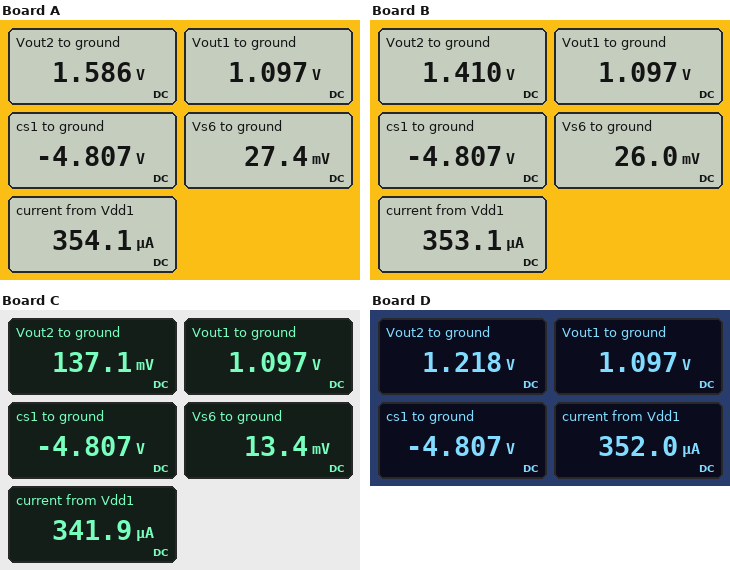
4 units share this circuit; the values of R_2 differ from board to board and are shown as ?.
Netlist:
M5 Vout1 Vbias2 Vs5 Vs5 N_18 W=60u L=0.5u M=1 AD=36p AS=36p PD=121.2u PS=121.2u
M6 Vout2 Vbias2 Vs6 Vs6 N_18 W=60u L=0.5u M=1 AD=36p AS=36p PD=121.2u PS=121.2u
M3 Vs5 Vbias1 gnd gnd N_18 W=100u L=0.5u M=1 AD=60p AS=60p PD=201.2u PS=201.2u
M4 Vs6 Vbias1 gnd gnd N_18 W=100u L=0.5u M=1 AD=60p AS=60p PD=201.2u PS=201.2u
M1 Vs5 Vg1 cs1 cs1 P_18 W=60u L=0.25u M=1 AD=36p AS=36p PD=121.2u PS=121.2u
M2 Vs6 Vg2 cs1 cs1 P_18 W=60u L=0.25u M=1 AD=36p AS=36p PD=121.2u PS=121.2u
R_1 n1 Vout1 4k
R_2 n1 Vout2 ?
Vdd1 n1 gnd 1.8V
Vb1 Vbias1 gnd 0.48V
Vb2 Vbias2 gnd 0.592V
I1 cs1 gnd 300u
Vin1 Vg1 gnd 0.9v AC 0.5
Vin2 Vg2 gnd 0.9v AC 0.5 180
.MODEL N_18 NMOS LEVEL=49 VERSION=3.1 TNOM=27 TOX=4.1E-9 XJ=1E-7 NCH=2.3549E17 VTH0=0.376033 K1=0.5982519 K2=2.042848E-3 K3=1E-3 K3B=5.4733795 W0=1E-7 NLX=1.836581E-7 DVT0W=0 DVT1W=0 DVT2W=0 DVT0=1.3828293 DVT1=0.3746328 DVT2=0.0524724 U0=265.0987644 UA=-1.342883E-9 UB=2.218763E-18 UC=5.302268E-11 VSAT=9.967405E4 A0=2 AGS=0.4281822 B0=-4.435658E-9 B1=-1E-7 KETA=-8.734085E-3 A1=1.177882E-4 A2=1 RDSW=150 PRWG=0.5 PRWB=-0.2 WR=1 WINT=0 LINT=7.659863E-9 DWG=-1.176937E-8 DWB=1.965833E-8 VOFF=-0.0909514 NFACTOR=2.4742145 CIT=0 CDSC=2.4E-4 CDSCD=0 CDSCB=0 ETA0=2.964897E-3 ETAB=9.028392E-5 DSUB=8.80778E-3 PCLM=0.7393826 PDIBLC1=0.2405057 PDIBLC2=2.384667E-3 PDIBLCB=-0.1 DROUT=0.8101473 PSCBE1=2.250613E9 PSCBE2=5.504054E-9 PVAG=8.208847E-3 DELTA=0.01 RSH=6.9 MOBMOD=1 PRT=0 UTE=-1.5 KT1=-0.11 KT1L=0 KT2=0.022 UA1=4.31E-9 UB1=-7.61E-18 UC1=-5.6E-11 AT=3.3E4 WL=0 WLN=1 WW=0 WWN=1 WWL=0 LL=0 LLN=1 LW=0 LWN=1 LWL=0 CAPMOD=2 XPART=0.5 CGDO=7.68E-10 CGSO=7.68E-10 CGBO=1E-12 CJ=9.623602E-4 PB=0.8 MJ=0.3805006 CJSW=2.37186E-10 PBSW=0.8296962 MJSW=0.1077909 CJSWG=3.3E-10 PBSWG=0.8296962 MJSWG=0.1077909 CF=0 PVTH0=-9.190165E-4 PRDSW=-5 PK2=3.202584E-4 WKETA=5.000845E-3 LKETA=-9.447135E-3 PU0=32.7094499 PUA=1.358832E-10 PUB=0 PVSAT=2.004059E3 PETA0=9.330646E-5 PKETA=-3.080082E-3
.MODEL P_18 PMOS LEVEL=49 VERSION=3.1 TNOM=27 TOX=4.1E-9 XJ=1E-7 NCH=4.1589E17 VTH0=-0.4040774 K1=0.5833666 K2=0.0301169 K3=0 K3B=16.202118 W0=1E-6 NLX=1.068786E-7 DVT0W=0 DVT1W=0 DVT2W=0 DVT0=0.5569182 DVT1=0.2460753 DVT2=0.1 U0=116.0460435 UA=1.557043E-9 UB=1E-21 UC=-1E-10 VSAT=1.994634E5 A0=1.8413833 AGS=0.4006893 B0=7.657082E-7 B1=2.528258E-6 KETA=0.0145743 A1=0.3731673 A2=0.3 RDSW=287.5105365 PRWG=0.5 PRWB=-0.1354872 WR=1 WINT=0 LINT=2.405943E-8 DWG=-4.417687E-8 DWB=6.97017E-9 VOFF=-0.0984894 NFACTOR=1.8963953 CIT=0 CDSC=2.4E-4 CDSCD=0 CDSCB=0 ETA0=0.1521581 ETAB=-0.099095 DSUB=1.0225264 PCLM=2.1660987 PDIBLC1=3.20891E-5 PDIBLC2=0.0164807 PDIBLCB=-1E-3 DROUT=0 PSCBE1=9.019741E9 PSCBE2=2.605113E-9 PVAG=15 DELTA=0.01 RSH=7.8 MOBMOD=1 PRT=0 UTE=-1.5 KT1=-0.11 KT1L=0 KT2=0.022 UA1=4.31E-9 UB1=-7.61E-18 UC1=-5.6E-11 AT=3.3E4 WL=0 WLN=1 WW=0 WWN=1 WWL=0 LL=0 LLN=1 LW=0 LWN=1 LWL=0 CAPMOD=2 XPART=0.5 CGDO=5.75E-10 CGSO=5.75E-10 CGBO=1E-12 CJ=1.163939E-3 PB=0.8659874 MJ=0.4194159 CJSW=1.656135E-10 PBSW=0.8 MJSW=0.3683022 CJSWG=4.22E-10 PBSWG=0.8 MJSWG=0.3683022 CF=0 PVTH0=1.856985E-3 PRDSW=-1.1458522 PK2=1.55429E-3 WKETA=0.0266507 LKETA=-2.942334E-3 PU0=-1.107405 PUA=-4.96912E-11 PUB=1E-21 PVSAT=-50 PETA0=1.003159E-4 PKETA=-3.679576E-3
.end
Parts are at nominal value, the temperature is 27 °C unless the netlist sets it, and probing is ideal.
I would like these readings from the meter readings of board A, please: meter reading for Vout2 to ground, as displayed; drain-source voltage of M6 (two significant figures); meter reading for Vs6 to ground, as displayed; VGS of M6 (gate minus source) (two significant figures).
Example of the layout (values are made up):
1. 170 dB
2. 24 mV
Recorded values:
1. 1.586 V
2. 1.6 V
3. 27.4 mV
4. 560 mV
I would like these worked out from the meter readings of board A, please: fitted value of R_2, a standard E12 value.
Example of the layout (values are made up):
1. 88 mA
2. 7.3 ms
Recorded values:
1. 1.2 kΩ
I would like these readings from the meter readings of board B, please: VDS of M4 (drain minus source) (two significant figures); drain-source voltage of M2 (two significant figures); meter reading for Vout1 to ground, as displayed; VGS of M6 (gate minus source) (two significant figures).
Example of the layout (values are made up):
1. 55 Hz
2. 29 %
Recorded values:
1. 26 mV
2. 4.8 V
3. 1.097 V
4. 570 mV
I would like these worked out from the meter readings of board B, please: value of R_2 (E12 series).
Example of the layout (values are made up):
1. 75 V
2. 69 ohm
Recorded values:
1. 2.2 kΩ
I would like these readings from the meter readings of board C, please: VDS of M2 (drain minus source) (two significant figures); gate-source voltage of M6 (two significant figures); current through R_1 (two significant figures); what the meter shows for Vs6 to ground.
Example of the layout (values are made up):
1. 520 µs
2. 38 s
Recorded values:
1. 4.8 V
2. 580 mV
3. 180 µA
4. 13.4 mV
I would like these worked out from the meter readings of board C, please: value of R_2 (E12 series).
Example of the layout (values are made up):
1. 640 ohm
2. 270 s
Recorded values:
1. 10 kΩ
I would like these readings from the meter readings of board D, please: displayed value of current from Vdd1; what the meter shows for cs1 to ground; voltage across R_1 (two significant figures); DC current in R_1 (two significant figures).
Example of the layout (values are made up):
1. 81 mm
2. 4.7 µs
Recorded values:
1. 352.0 µA
2. -4.807 V
3. 700 mV
4. 180 µA
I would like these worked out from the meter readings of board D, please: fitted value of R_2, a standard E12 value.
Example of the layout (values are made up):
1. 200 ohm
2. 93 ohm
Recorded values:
1. 3.3 kΩ
